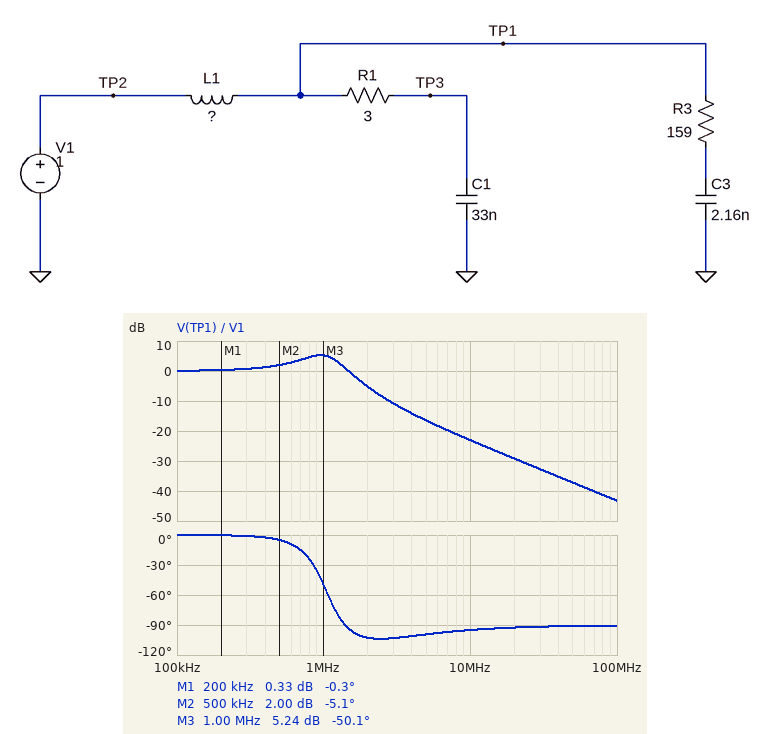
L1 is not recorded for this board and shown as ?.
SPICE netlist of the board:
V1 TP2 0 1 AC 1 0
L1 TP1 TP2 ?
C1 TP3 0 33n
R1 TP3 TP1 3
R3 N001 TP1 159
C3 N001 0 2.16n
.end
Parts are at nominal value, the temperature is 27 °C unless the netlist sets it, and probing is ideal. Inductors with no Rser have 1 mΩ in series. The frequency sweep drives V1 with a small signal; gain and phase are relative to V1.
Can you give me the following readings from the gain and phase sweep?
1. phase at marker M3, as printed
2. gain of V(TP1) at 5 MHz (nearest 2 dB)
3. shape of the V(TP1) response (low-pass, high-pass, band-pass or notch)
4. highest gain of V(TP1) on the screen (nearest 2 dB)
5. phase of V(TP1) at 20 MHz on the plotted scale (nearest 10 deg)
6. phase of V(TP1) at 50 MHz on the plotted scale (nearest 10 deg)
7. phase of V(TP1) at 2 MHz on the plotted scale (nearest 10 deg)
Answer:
-50.1 deg
-16 dB
low-pass
6 dB
-90 deg
-90 deg
-100 deg
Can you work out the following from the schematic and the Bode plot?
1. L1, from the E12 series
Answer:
680 nH
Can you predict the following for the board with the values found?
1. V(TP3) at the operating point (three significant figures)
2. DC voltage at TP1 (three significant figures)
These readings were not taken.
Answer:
1.00 V
1.00 V
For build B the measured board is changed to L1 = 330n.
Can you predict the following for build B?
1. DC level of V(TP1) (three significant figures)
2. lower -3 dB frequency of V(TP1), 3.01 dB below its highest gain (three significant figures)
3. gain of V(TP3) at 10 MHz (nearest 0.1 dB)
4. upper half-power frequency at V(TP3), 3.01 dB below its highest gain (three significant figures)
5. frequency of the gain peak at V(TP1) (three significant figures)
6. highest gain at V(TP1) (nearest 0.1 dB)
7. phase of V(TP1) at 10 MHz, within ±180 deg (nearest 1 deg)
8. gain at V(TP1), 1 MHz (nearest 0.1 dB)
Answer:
1.00 V
362 kHz
-32.7 dB
1.77 MHz
1.30 MHz
3.5 dB
-91 deg
2.9 dB
